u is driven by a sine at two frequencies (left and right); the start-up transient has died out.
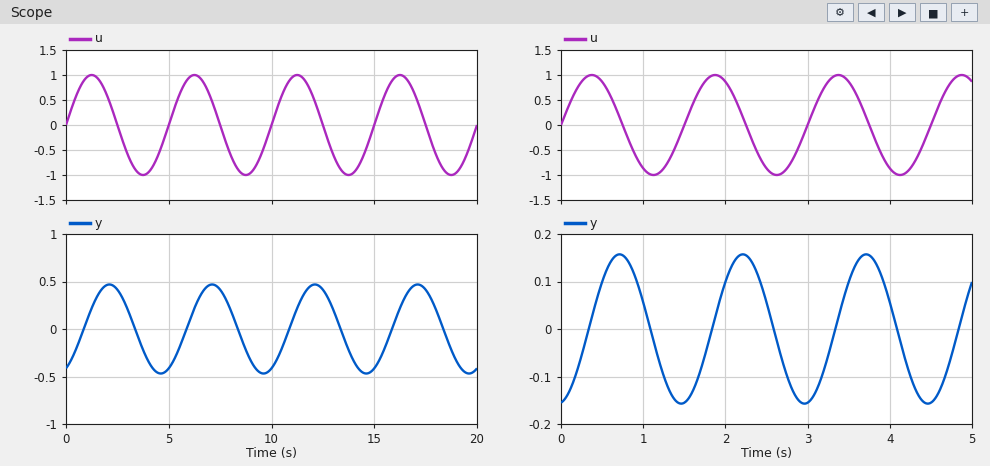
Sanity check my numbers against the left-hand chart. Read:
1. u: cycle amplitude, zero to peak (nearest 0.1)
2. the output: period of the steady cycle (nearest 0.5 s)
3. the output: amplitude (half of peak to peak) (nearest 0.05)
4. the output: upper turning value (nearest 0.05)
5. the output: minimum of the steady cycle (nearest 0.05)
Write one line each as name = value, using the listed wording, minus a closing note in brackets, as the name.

u: cycle amplitude, zero to peak = 1.0
the output: period of the steady cycle = 5.0 s
the output: amplitude (half of peak to peak) = 0.45
the output: upper turning value = 0.45
the output: minimum of the steady cycle = -0.45
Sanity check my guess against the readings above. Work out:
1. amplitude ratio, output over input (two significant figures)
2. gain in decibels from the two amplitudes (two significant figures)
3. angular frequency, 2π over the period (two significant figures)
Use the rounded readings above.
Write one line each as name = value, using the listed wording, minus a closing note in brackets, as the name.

amplitude ratio, output over input = 0.45
gain in decibels from the two amplitudes = -6.9 dB
angular frequency, 2π over the period = 1.3 rad/s
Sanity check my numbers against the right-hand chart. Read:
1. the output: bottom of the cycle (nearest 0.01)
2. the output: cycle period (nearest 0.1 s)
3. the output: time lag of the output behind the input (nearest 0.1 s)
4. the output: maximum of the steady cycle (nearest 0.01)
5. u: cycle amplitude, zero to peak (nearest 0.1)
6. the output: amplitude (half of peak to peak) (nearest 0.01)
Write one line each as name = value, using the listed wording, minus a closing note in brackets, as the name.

the output: bottom of the cycle = -0.16
the output: cycle period = 1.5 s
the output: time lag of the output behind the input = 0.3 s
the output: maximum of the steady cycle = 0.16
u: cycle amplitude, zero to peak = 1.0
the output: amplitude (half of peak to peak) = 0.16
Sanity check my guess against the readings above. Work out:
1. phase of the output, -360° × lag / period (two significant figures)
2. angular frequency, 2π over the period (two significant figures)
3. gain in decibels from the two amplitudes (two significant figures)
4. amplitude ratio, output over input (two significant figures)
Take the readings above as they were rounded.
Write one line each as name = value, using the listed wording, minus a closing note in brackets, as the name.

phase of the output, -360° × lag / period = -72°
angular frequency, 2π over the period = 4.2 rad/s
gain in decibels from the two amplitudes = -16 dB
amplitude ratio, output over input = 0.16
